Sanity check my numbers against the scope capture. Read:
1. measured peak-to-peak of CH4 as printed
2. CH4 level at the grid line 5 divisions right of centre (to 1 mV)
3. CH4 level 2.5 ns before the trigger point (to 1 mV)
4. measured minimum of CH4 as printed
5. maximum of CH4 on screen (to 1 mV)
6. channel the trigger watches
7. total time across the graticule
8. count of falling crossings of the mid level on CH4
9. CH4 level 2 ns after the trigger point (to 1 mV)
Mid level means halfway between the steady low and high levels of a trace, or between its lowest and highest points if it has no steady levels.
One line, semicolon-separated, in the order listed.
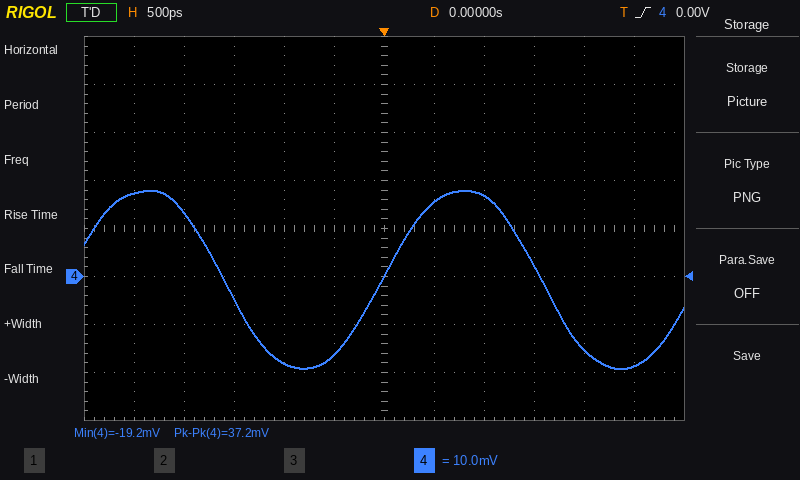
37.2 mV; -19 mV; 17 mV; -19.2 mV; 18 mV; CH4; 6 ns; 2; -15 mV
